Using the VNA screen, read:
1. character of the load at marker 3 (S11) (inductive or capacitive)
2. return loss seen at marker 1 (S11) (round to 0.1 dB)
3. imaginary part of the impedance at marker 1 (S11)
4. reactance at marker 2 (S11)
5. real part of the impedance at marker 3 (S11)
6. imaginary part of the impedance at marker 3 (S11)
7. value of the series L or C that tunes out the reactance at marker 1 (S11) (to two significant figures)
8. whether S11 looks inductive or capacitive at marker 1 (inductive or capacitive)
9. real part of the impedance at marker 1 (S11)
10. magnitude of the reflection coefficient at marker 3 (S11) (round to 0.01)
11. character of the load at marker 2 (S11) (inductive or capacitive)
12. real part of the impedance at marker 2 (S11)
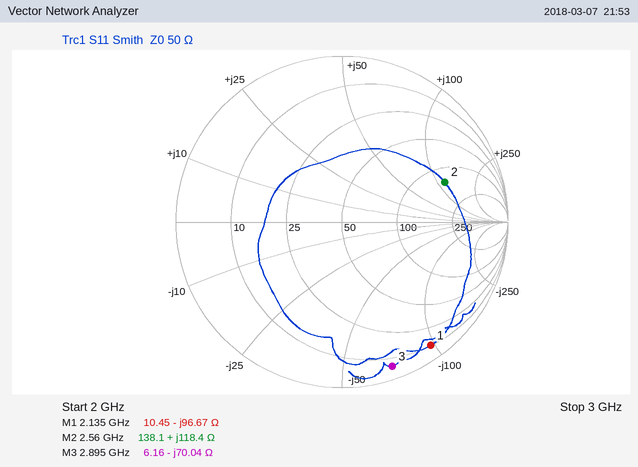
capacitive
0.8 dB
-96.67 Ω
+118.4 Ω
6.16 Ω
-70.04 Ω
7.2 nH
capacitive
10.45 Ω
0.92
inductive
138.1 Ω
